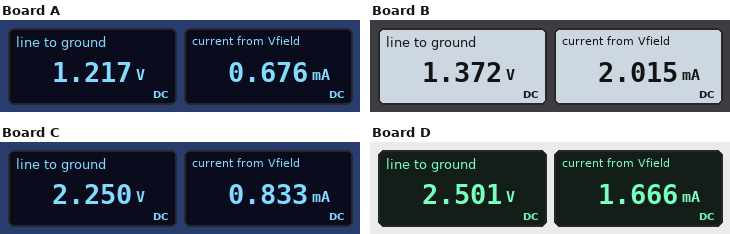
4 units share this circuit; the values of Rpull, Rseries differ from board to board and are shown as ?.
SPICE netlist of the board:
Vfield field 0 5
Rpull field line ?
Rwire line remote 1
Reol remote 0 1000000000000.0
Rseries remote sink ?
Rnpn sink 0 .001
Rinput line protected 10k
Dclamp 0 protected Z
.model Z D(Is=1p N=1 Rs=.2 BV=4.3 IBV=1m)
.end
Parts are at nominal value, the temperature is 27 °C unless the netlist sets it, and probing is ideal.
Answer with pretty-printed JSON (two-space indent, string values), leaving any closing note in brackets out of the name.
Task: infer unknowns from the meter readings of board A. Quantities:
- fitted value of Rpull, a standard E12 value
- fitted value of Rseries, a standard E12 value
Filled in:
{
  "fitted value of Rpull, a standard E12 value": "5.6 kΩ",
  "fitted value of Rseries, a standard E12 value": "1.8 kΩ"
}
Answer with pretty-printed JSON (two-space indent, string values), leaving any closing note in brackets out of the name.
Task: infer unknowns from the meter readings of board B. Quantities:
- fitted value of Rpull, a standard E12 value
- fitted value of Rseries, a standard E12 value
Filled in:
{
  "fitted value of Rpull, a standard E12 value": "1.8 kΩ",
  "fitted value of Rseries, a standard E12 value": "680 Ω"
}
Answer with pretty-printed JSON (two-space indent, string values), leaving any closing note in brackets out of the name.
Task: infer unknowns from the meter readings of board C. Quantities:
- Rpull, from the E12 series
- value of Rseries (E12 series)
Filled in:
{
  "Rpull, from the E12 series": "3.3 kΩ",
  "value of Rseries": "2.7 kΩ"
}
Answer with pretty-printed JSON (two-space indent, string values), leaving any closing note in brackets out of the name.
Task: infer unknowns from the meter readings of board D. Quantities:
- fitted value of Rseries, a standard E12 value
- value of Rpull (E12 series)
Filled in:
{
  "fitted value of Rseries, a standard E12 value": "1.5 kΩ",
  "value of Rpull": "1.5 kΩ"
}
